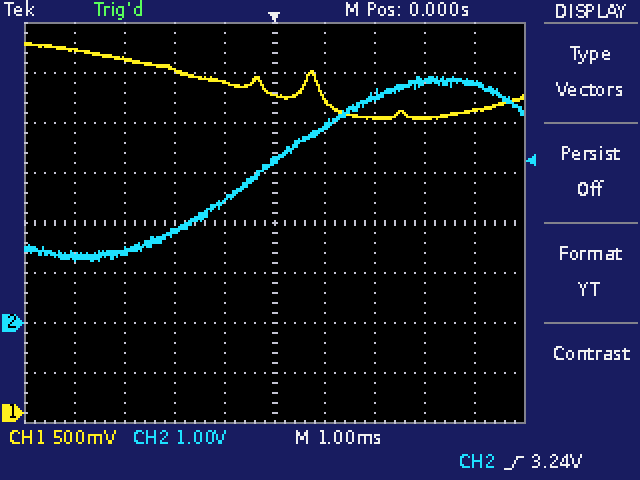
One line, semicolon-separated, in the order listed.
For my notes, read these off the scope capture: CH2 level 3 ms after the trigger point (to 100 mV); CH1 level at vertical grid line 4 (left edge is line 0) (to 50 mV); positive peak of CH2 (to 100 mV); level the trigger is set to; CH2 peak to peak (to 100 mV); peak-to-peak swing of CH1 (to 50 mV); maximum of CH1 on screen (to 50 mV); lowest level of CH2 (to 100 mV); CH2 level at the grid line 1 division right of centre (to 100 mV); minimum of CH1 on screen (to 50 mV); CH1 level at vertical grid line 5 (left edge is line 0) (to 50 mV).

4.8 V; 3.30 V; 4.9 V; 3.24 V; 3.7 V; 750 mV; 3.70 V; 1.2 V; 3.9 V; 2.95 V; 3.20 V
